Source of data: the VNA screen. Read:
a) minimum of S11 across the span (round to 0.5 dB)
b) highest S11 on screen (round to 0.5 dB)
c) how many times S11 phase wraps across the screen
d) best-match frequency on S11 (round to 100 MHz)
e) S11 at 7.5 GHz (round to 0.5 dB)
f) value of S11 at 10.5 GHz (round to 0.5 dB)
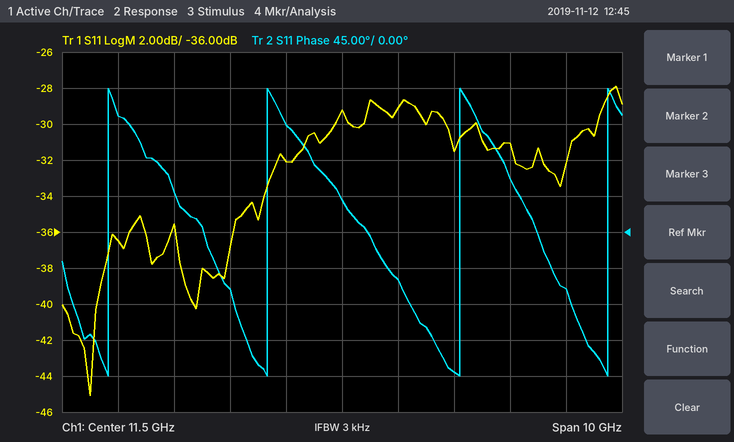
-45.0 dB
-28.0 dB
4
7.0 GHz
-36.5 dB
-32.0 dB
